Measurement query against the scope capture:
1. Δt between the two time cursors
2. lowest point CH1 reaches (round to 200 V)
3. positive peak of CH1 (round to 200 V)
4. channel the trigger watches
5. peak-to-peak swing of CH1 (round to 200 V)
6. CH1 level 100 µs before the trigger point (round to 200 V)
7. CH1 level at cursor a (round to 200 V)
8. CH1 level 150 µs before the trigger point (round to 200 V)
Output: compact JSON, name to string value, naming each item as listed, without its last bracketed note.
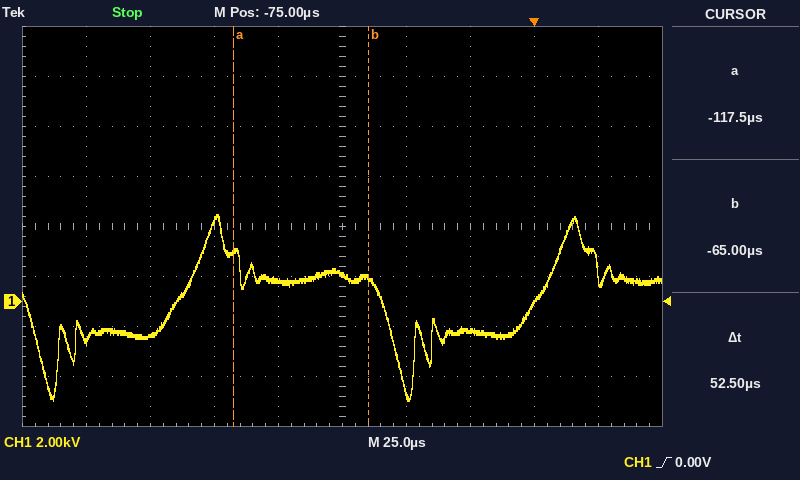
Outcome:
{"Δt between the two time cursors": "52.5 µs", "lowest point CH1 reaches": "-4.0 kV", "positive peak of CH1": "3.4 kV", "channel the trigger watches": "CH1", "peak-to-peak swing of CH1": "7.4 kV", "CH1 level 100 µs before the trigger point": "800 V", "CH1 level at cursor a": "2.0 kV", "CH1 level 150 µs before the trigger point": "-1.4 kV"}
